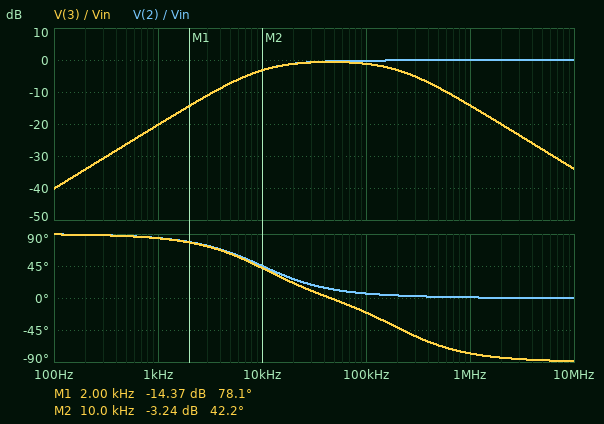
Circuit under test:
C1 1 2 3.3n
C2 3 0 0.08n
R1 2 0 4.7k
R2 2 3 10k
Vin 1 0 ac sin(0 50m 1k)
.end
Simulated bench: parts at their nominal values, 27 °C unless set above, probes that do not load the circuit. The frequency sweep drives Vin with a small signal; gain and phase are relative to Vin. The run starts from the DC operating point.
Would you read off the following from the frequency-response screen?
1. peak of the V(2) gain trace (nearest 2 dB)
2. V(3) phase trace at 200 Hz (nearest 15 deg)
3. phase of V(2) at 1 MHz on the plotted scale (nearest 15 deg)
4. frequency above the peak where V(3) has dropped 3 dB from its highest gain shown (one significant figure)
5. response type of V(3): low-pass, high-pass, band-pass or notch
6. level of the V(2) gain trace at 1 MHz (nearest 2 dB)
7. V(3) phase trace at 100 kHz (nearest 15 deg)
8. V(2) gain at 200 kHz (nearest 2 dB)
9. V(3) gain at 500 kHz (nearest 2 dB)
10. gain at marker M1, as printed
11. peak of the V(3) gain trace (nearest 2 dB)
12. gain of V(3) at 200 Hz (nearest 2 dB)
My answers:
0 dB
90 deg
0 deg
200 kHz
band-pass
0 dB
-15 deg
0 dB
-8 dB
-14.37 dB
0 dB
-34 dB
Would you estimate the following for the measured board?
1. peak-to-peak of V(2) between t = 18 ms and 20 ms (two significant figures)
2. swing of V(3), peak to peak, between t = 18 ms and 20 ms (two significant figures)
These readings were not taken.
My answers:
9.7 mV
9.7 mV
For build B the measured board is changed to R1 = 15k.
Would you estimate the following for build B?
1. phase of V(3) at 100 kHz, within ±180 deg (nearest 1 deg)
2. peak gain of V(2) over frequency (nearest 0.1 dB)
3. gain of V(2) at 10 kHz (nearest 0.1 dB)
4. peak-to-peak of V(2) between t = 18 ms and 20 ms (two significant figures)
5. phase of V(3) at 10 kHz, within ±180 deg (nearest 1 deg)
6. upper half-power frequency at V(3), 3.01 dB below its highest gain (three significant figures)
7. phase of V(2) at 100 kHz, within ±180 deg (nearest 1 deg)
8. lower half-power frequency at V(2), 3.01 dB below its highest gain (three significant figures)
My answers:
-24 deg
0 dB
-0.6 dB
30 mV
15 deg
210 kHz
2 deg
3.30 kHz
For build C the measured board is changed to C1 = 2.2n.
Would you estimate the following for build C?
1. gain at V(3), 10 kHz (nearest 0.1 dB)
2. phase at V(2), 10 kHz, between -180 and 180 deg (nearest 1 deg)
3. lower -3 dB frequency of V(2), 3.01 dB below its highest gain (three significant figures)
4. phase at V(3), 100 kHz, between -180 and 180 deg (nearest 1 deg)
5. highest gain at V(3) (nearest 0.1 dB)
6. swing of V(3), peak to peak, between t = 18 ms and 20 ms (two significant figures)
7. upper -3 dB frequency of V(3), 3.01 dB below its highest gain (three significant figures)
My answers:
-5.4 dB
56 deg
16.0 kHz
-17 deg
-0.9 dB
6.5 mV
235 kHz
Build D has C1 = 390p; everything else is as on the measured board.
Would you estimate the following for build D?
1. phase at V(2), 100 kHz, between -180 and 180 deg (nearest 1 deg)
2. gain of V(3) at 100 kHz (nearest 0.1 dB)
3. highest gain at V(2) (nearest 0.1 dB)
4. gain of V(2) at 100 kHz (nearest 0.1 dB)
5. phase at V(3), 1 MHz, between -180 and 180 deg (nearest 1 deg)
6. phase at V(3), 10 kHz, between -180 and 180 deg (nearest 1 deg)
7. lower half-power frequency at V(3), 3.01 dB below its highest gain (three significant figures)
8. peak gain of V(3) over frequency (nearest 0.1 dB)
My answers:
39 deg
-4.5 dB
0 dB
-3.5 dB
-72 deg
79 deg
46.3 kHz
-4.3 dB
